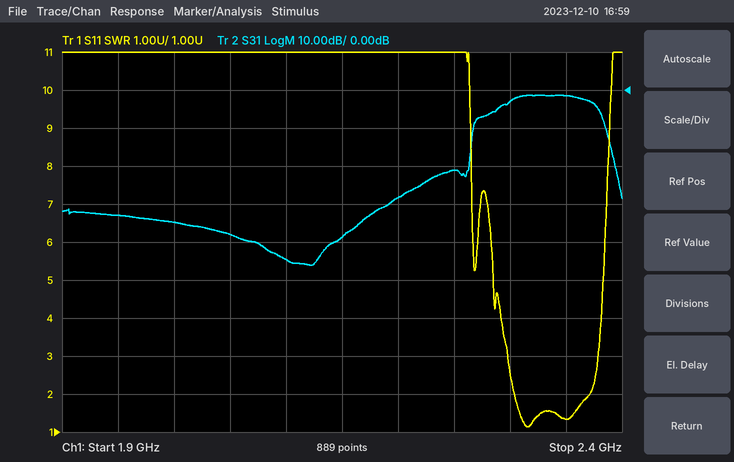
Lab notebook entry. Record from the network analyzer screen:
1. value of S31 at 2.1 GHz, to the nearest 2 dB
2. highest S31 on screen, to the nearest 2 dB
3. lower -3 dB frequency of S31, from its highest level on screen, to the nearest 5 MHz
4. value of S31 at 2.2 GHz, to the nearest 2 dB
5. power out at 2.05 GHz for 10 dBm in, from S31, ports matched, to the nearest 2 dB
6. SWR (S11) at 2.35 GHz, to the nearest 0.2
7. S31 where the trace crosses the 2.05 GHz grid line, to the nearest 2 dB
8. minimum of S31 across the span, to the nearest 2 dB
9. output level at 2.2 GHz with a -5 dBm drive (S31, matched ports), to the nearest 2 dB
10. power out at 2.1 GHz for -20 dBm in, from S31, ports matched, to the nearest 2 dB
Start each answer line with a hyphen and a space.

- -44 dB
- -2 dB
- 2.290 GHz
- -28 dB
- -28 dBm
- 1.4
- -38 dB
- -46 dB
- -34 dBm
- -64 dBm
